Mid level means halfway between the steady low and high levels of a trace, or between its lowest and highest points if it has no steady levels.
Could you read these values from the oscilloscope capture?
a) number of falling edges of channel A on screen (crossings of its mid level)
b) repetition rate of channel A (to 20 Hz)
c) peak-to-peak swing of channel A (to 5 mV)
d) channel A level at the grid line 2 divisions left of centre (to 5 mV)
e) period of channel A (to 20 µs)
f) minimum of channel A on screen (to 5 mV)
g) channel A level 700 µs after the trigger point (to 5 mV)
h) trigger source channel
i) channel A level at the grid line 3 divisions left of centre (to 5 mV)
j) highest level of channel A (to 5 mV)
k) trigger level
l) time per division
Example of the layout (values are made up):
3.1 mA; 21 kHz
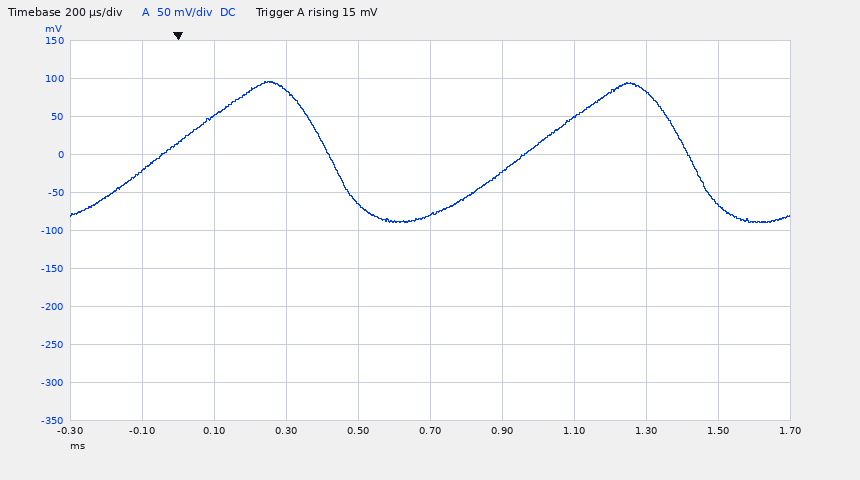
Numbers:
2; 1.00 kHz; 185 mV; 85 mV; 1.00 ms; -90 mV; -80 mV; channel A; 50 mV; 95 mV; 15 mV; 200 µs
